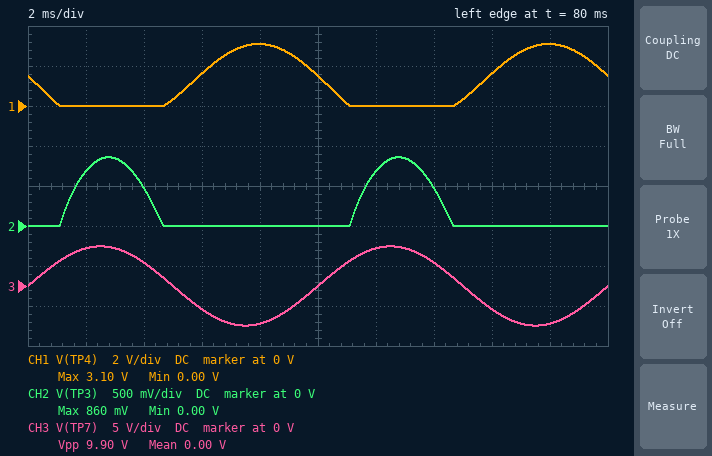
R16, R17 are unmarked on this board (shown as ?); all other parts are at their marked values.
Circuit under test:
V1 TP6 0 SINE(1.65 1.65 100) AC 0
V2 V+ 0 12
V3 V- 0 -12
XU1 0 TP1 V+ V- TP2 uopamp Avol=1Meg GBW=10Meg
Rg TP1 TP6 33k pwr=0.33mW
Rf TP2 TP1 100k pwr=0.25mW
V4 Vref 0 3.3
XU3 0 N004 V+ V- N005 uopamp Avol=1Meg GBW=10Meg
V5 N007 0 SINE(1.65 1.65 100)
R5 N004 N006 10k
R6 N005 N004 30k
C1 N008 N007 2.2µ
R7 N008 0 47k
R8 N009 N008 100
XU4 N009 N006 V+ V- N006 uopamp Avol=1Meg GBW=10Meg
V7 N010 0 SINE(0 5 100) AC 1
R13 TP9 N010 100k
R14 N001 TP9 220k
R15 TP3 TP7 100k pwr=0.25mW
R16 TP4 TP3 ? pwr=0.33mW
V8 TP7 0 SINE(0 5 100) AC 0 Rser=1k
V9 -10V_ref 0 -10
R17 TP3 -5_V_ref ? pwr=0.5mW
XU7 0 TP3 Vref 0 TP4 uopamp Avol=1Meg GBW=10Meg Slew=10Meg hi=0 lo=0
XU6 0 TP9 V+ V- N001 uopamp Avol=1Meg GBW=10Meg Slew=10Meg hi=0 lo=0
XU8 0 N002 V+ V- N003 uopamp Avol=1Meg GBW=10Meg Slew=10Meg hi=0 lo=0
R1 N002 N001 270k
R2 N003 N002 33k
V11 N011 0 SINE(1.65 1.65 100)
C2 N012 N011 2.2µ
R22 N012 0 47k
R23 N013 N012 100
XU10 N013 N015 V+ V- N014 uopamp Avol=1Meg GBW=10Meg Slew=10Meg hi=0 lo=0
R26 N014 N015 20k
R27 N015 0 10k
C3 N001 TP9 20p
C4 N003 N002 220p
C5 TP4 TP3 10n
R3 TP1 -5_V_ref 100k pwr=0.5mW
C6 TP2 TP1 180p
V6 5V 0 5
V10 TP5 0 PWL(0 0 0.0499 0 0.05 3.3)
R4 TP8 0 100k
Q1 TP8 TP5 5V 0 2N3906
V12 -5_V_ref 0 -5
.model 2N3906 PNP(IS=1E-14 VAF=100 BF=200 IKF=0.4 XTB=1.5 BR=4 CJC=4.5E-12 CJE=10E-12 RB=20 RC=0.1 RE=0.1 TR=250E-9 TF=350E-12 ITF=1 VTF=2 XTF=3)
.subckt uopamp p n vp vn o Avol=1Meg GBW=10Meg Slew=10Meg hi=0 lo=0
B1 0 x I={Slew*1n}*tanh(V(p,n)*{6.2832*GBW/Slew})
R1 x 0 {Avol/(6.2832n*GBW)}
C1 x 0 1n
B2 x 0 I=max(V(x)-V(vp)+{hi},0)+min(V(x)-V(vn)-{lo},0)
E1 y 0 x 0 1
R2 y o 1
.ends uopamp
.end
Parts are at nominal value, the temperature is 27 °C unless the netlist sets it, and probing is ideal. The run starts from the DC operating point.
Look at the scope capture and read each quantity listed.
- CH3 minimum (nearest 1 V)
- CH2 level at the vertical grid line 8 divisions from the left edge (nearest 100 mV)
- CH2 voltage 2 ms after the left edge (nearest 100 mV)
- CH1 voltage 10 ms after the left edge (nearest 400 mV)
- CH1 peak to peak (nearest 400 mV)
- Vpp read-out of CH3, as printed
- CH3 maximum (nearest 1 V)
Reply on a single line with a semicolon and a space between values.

-5 V; 0 V; 700 mV; 1.6 V; 3.2 V; 9.90 V; 5 V
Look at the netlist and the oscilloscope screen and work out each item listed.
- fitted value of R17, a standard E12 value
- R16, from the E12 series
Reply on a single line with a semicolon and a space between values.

270 kΩ; 47 kΩ
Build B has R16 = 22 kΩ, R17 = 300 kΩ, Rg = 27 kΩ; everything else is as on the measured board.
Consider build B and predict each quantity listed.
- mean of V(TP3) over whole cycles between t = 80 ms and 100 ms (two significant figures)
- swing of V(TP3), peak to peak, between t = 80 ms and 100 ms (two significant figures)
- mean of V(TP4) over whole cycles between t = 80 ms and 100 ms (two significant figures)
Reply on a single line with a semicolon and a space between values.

140 mV; 550 mV; 540 mV
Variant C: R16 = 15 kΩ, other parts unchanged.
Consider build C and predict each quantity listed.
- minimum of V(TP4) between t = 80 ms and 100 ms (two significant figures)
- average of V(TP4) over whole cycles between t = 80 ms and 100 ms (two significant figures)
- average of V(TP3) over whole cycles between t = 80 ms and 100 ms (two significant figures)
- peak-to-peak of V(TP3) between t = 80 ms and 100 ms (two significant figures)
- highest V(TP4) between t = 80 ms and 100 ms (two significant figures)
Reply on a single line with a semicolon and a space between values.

-9.8 mV; 390 mV; 92 mV; 380 mV; 1.0 V
